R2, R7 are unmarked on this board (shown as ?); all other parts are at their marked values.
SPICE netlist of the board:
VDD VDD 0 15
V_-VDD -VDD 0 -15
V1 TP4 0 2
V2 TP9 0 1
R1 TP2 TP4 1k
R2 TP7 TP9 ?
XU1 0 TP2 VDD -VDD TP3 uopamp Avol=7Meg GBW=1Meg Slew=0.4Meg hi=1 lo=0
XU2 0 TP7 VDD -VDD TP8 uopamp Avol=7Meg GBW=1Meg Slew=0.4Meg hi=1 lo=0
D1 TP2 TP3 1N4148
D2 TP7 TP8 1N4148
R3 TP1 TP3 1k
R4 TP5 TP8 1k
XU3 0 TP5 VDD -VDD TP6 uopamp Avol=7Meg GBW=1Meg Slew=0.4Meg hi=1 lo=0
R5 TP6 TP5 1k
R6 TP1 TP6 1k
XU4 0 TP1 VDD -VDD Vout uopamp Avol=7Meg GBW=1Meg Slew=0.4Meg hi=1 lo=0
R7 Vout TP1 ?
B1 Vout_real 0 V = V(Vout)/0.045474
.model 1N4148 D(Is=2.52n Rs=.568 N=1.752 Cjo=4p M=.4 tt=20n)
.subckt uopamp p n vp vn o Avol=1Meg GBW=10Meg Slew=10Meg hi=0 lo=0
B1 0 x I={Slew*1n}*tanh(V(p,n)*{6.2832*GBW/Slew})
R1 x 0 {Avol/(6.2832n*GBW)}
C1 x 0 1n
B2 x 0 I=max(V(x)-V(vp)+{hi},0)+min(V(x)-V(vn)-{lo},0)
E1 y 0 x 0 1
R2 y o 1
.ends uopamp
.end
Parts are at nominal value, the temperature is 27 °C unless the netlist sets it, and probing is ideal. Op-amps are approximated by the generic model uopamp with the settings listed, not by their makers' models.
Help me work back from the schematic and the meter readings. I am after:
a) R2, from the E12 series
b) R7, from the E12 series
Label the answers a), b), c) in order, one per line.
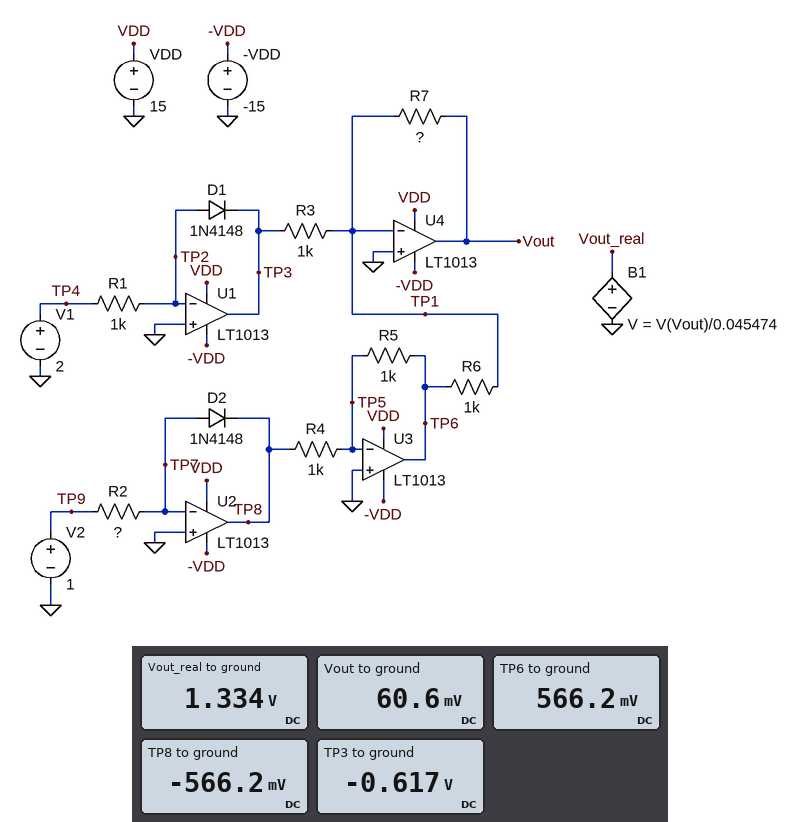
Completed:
a) 1.5 kΩ
b) 1.2 kΩ
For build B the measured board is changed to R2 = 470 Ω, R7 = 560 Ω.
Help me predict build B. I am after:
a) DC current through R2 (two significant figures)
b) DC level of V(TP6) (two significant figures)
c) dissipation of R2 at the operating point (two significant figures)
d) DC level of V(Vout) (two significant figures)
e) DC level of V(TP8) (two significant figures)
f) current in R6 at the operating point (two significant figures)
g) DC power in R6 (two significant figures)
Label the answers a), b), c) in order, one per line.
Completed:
a) 2.1 mA
b) 620 mV
c) 2.1 mW
d) -1.6 mV
e) -620 mV
f) 620 µA
g) 380 µW
